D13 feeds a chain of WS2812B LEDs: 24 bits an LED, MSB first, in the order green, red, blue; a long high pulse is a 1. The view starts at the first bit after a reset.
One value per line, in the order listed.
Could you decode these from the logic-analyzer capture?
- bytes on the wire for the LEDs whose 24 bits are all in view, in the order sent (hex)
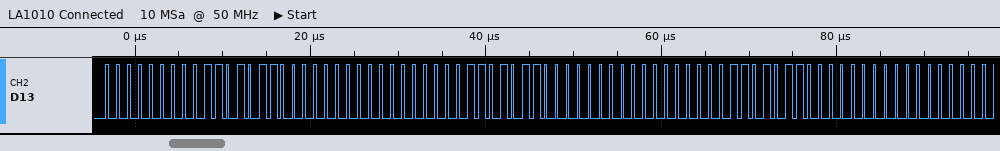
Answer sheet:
00 6B 00 00 6B 00 00 6B 00
